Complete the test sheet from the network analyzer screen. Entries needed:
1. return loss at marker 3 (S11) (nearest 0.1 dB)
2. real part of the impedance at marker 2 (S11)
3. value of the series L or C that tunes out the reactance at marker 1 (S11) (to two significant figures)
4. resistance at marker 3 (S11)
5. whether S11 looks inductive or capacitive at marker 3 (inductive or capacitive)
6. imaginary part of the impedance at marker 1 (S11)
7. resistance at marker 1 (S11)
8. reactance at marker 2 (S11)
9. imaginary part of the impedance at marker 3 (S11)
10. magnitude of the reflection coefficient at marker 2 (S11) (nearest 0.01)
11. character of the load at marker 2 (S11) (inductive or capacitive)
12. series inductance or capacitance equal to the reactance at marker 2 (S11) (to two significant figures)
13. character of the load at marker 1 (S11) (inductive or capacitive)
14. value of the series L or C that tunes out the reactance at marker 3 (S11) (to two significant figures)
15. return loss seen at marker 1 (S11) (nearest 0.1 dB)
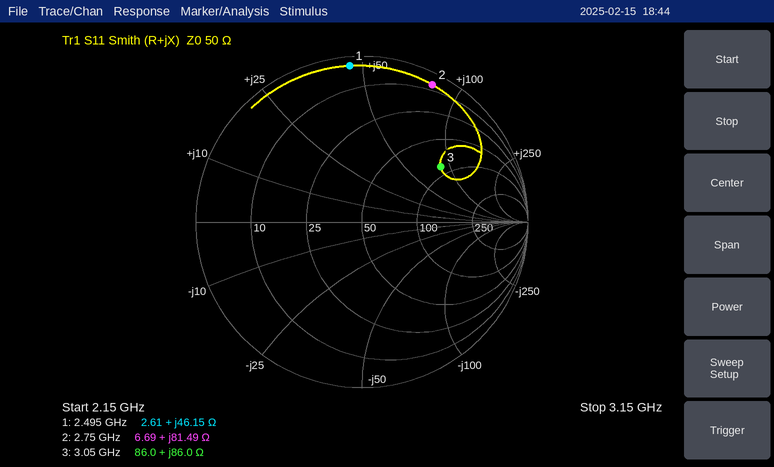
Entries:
4.7 dB
6.69 Ω
1.4 pF
86.0 Ω
inductive
+46.15 Ω
2.61 Ω
+81.49 Ω
+86.0 Ω
0.93
inductive
4.7 nH
inductive
610 fF
0.5 dB
